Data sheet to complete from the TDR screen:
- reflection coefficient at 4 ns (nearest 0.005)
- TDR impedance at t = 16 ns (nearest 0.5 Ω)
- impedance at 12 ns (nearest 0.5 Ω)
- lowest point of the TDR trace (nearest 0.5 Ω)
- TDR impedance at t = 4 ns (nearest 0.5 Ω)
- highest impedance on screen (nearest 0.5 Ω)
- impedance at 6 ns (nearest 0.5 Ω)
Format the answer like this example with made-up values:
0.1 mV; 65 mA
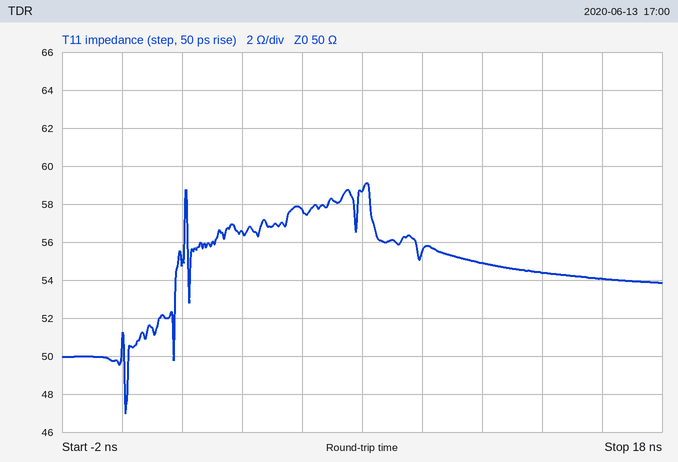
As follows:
+0.060; 54.0 Ω; 55.0 Ω; 47.0 Ω; 56.5 Ω; 59.0 Ω; 57.5 Ω
